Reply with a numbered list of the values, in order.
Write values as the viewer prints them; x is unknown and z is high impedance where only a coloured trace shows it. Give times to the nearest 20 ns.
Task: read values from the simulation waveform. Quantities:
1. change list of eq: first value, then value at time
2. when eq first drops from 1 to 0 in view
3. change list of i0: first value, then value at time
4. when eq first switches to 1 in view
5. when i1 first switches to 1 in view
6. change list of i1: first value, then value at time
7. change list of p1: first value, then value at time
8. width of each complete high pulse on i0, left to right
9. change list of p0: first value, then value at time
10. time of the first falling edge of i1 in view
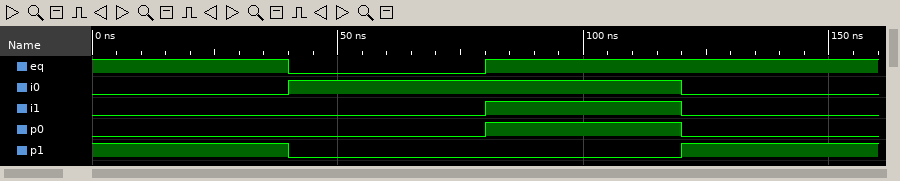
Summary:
1. 1, 0 at 40 ns, 1 at 80 ns
2. 40 ns
3. 0, 1 at 40 ns, 0 at 120 ns
4. 80 ns
5. 80 ns
6. 0, 1 at 80 ns, 0 at 120 ns
7. 1, 0 at 40 ns, 1 at 120 ns
8. 80 ns
9. 0, 1 at 80 ns, 0 at 120 ns
10. 120 ns
